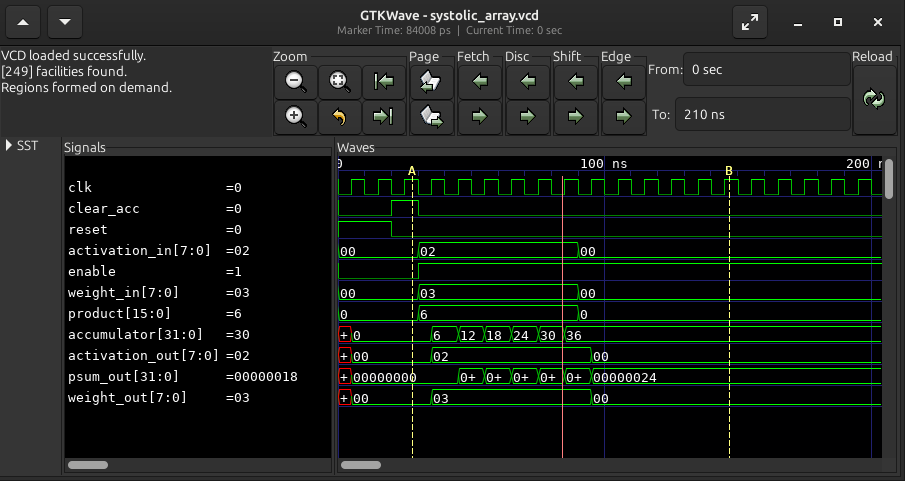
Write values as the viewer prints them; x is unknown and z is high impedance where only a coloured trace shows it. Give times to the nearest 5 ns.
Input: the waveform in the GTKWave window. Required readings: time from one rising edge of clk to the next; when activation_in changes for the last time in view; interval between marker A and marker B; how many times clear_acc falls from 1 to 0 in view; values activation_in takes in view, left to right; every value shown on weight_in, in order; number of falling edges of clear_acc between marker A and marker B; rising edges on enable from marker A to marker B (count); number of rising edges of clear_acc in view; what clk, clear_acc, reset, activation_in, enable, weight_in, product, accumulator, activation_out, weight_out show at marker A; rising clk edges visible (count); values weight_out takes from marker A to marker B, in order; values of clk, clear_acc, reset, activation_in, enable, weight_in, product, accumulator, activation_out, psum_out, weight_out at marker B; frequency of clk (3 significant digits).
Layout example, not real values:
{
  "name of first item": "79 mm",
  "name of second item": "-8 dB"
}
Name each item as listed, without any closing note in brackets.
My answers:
{
  "time from one rising edge of clk to the next": "10 ns",
  "when activation_in changes for the last time in view": "90 ns",
  "interval between marker A and marker B": "120 ns",
  "how many times clear_acc falls from 1 to 0 in view": "1",
  "values activation_in takes in view, left to right": "00, 02, 00",
  "every value shown on weight_in, in order": "00, 03, 00",
  "number of falling edges of clear_acc between marker A and marker B": "1",
  "rising edges on enable from marker A to marker B": "1",
  "number of rising edges of clear_acc in view": "1",
  "what clk, clear_acc, reset, activation_in, enable, weight_in, product, accumulator, activation_out, weight_out show at marker A": "clk=1, clear_acc=1, reset=0, activation_in=00, enable=0, weight_in=00, product=0, accumulator=0, activation_out=00, weight_out=00",
  "rising clk edges visible": "20",
  "values weight_out takes from marker A to marker B, in order": "00, 03, 00",
  "values of clk, clear_acc, reset, activation_in, enable, weight_in, product, accumulator, activation_out, psum_out, weight_out at marker B": "clk=1, clear_acc=0, reset=0, activation_in=00, enable=1, weight_in=00, product=0, accumulator=36, activation_out=00, psum_out=00000024, weight_out=00",
  "frequency of clk": "100 MHz"
}
